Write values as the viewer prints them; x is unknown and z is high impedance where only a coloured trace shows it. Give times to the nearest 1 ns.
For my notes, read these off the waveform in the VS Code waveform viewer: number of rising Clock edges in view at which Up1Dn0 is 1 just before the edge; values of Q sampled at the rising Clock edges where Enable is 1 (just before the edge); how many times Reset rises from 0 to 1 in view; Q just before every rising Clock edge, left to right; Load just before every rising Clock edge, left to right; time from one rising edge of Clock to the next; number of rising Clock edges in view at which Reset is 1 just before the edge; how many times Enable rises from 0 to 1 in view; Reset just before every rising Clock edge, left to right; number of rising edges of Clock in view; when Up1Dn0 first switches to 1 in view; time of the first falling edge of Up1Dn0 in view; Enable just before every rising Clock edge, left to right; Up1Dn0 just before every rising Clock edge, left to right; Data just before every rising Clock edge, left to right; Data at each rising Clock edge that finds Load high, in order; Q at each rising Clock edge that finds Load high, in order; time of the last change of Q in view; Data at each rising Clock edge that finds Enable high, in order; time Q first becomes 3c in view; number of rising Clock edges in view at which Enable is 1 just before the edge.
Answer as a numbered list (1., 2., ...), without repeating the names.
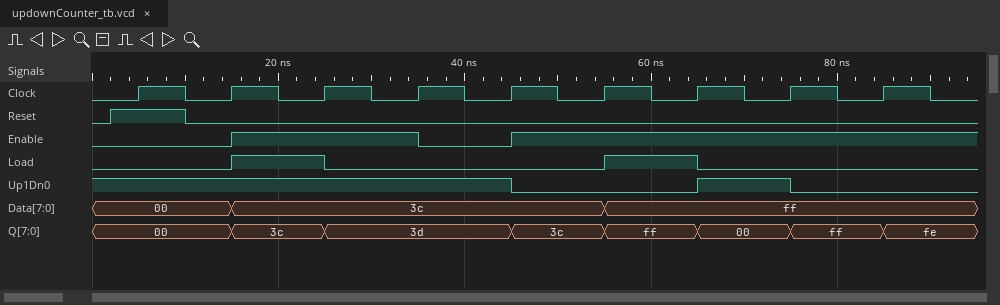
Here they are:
1. 6
2. 3c, 3d, 3c, ff, 00, ff
3. 1
4. 00, 00, 3c, 3d, 3d, 3c, ff, 00, ff
5. 0 0 1 0 0 0 1 0 0
6. 10 ns
7. 1
8. 2
9. 1 0 0 0 0 0 0 0 0
10. 9
11. 65 ns
12. 45 ns
13. 0 0 1 1 0 1 1 1 1
14. 1 1 1 1 1 0 0 1 0
15. 00, 00, 3c, 3c, 3c, 3c, ff, ff, ff
16. 3c, ff
17. 3c, ff
18. 85 ns
19. 3c, 3c, 3c, ff, ff, ff
20. 15 ns
21. 6
